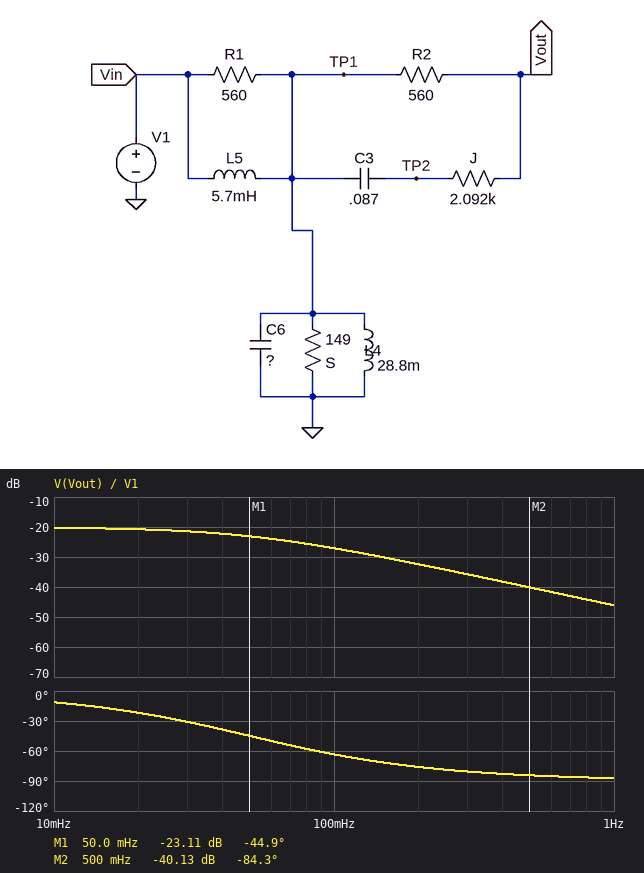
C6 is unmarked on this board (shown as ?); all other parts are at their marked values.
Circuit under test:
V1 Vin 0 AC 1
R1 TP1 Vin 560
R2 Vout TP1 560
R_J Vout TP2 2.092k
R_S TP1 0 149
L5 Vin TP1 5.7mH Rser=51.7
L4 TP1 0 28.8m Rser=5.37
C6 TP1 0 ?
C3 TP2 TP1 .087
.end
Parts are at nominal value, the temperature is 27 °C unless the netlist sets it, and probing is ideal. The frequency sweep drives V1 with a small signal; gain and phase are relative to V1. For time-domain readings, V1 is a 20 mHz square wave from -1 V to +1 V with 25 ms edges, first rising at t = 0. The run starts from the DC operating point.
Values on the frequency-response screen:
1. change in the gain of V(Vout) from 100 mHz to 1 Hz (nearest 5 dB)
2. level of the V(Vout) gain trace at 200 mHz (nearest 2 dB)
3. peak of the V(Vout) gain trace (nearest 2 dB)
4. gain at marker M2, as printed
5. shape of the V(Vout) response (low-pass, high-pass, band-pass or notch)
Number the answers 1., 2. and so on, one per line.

1. -20 dB
2. -32 dB
3. -20 dB
4. -40.13 dB
5. low-pass
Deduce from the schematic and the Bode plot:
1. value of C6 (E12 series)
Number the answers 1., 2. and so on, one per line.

1. 680 mF
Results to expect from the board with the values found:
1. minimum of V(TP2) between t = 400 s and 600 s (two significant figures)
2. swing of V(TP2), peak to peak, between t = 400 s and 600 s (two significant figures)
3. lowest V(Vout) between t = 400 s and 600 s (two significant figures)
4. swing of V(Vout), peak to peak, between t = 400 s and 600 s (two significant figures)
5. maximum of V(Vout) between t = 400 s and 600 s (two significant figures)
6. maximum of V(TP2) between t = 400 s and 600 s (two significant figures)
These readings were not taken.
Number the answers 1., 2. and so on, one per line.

1. -99 mV
2. 200 mV
3. -99 mV
4. 200 mV
5. 99 mV
6. 99 mV
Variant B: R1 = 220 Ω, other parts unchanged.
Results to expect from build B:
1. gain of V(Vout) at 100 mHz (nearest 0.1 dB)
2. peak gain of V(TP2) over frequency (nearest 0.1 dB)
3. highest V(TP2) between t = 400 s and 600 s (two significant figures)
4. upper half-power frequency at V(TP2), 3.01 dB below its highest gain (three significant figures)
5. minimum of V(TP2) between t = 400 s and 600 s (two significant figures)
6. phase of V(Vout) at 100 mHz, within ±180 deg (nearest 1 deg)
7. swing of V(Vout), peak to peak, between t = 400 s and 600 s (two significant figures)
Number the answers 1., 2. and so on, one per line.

1. -26.0 dB
2. -19.2 dB
3. 110 mV
4. 50.8 mHz
5. -110 mV
6. -63 deg
7. 220 mV
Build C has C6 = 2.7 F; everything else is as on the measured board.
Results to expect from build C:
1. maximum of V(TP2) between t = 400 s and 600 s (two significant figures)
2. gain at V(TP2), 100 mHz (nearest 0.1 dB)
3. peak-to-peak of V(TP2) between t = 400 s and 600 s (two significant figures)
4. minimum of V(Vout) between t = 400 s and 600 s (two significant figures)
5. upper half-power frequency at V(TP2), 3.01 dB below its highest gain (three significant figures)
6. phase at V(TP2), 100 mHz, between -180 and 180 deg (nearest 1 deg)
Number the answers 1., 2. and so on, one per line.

1. 75 mV
2. -38.2 dB
3. 150 mV
4. -75 mV
5. 12.6 mHz
6. -83 deg
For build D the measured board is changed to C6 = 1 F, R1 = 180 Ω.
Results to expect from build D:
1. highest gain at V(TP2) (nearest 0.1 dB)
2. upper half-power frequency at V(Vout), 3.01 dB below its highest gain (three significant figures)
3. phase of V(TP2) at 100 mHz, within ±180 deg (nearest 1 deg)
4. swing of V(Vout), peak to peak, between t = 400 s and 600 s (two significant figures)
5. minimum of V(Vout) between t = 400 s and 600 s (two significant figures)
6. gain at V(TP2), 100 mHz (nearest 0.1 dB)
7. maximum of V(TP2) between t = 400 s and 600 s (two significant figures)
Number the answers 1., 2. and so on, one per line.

1. -18.8 dB
2. 34.7 mHz
3. -71 deg
4. 230 mV
5. -110 mV
6. -28.5 dB
7. 110 mV
